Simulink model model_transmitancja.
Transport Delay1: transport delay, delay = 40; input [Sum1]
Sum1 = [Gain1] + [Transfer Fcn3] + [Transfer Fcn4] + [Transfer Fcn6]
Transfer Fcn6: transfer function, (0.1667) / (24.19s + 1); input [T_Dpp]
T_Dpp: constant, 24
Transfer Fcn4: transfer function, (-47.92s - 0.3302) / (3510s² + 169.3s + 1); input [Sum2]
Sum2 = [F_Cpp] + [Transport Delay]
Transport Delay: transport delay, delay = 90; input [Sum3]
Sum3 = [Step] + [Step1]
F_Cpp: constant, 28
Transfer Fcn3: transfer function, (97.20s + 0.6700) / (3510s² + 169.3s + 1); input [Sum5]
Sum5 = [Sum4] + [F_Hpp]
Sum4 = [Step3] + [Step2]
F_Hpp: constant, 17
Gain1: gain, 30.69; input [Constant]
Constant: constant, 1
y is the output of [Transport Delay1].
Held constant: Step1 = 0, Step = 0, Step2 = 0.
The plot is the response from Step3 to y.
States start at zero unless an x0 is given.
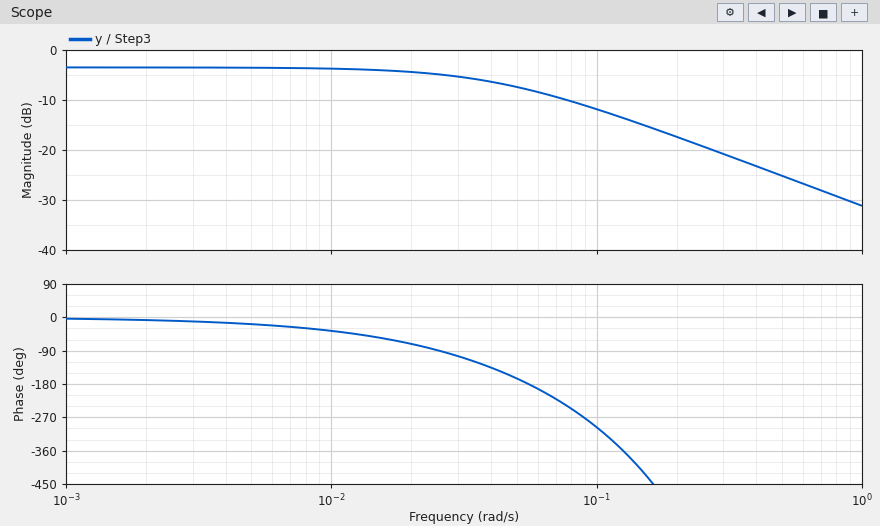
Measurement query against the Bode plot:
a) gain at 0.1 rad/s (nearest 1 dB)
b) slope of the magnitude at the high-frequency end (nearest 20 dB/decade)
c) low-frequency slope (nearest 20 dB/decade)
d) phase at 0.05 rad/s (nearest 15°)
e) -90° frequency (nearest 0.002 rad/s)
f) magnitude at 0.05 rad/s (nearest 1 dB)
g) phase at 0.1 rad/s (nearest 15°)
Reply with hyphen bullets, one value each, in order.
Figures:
- -12 dB
- -20 dB/decade
- 0 dB/decade
- -165°
- 0.026 rad/s
- -7 dB
- -300°
